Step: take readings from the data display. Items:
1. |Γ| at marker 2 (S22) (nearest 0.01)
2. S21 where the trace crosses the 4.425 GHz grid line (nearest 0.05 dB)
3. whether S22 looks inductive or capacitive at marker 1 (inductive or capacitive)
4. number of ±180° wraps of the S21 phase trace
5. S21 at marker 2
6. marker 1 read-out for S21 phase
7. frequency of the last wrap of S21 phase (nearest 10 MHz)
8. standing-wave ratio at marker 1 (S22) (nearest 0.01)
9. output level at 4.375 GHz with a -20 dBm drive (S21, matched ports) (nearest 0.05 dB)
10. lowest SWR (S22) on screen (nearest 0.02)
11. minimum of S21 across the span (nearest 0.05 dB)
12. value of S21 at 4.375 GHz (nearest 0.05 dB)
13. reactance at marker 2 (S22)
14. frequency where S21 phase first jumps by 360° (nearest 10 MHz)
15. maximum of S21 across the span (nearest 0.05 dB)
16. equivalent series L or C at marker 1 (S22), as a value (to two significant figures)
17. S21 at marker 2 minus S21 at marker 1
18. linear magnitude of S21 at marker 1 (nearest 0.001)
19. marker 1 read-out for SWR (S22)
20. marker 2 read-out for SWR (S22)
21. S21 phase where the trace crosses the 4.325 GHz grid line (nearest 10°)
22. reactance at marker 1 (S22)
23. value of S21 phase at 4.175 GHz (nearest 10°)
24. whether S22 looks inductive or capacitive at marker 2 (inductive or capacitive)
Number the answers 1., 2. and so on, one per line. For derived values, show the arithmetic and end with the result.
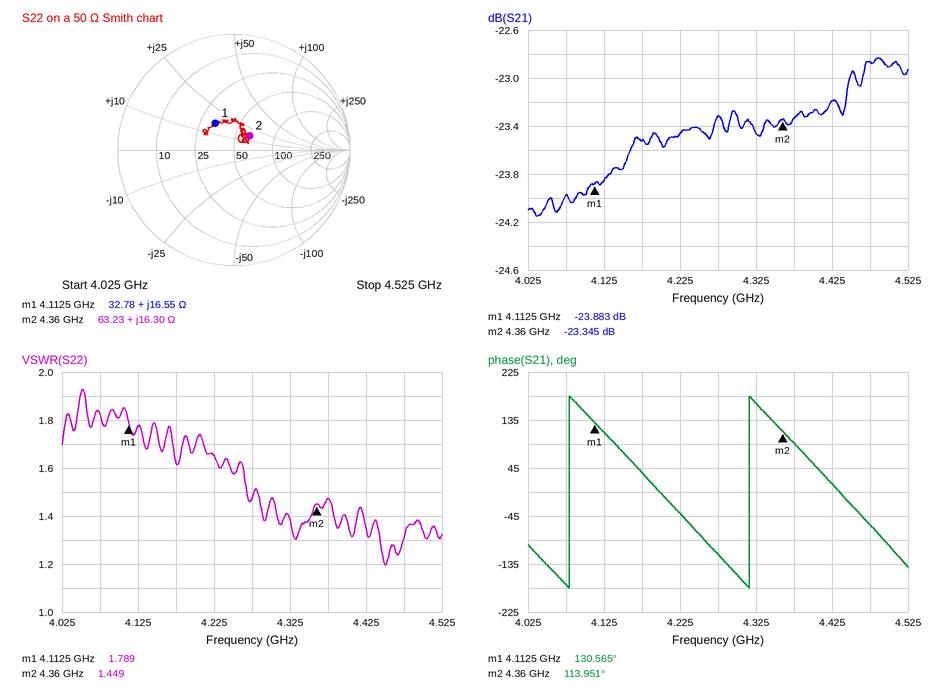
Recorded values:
1. 0.18
2. -23.20 dB
3. inductive
4. 2
5. -23.345 dB
6. 130.565°
7. 4.32 GHz
8. 1.79
9. -20 dBm + (-23.35 dB) = -43.35 dBm
10. 1.20
11. -24.15 dB
12. -23.35 dB
13. +16.30 Ω
14. 4.08 GHz
15. -22.85 dB
16. L = 16.55 Ω/(2π × 4.1125 GHz) ≈ 640 pH
17. -23.345 − (-23.883) = 0.538 dB
18. 10^(-23.883/20) ≈ 0.064
19. 1.789
20. 1.449
21. 170°
22. +16.55 Ω
23. 40°
24. inductive
